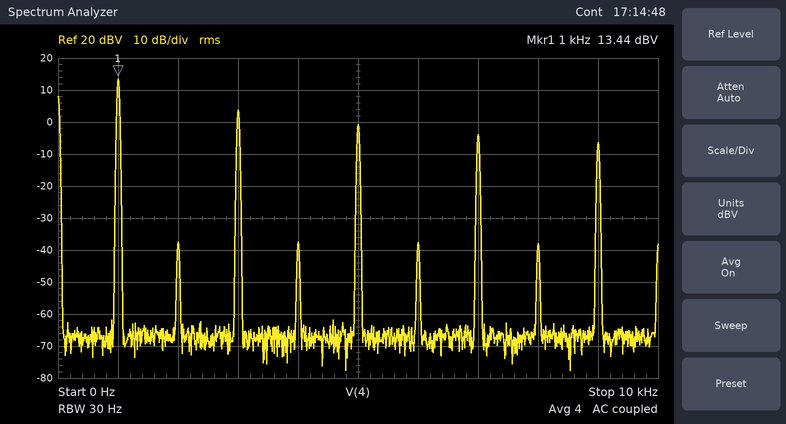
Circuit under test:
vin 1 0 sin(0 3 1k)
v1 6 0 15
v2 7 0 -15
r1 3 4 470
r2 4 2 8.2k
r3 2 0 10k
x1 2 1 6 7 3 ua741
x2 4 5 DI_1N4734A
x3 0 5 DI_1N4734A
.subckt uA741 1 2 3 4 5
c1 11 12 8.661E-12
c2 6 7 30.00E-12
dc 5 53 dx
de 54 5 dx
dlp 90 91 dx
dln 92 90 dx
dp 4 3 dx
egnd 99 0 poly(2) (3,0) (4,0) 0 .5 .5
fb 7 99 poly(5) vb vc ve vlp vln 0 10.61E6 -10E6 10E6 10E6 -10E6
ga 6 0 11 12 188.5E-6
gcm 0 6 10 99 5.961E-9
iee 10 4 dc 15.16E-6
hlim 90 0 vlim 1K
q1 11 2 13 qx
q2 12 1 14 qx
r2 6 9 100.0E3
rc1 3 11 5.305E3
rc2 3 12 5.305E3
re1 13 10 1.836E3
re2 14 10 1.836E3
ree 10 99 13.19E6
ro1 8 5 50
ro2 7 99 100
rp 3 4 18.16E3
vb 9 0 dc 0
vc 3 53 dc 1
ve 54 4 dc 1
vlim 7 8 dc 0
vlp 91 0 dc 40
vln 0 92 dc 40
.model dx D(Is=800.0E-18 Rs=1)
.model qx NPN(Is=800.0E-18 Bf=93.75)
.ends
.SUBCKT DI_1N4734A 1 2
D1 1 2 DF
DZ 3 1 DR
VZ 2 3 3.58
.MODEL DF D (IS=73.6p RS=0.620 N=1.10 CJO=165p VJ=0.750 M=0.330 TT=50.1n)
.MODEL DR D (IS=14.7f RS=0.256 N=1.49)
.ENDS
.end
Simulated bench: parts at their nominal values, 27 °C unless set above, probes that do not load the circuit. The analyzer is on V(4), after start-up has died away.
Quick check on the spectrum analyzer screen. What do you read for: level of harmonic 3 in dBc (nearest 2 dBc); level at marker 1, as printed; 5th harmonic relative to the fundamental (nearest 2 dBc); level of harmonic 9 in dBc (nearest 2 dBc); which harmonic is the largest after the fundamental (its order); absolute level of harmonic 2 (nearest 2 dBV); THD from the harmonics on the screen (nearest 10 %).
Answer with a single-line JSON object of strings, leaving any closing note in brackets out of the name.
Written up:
{"level of harmonic 3 in dBc": "-10 dBc", "level at marker 1, as printed": "13.44 dBV", "5th harmonic relative to the fundamental": "-14 dBc", "level of harmonic 9 in dBc": "-20 dBc", "which harmonic is the largest after the fundamental": "3", "absolute level of harmonic 2": "-38 dBV", "THD from the harmonics on the screen": "40 %"}
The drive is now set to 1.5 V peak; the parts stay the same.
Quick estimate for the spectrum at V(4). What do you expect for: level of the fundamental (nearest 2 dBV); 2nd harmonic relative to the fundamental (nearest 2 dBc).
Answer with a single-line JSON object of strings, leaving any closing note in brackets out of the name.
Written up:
{"level of the fundamental": "-118 dBV", "2nd harmonic relative to the fundamental": "-54 dBc"}
